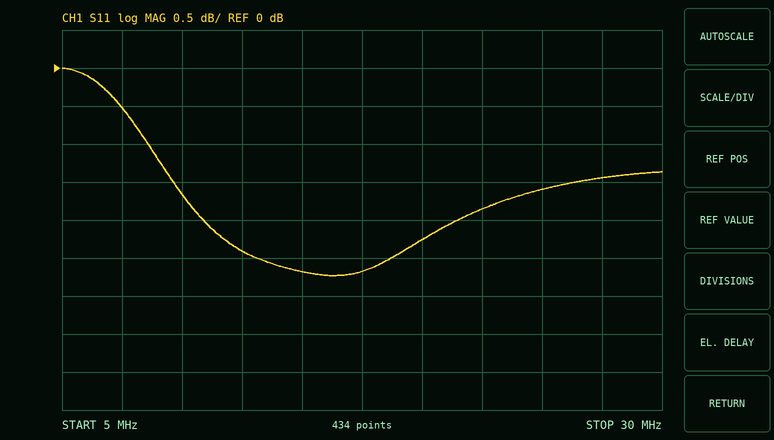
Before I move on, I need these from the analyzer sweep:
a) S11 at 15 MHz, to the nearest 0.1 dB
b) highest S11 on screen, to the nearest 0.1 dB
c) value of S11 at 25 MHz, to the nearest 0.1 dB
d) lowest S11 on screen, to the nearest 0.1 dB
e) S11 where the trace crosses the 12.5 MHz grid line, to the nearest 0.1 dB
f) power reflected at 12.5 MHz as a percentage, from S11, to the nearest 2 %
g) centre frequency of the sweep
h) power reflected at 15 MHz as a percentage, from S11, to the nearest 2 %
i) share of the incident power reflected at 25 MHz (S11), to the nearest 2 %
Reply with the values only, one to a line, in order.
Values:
-2.7 dB
0.0 dB
-1.6 dB
-2.7 dB
-2.4 dB
58 %
17.5 MHz
54 %
70 %
